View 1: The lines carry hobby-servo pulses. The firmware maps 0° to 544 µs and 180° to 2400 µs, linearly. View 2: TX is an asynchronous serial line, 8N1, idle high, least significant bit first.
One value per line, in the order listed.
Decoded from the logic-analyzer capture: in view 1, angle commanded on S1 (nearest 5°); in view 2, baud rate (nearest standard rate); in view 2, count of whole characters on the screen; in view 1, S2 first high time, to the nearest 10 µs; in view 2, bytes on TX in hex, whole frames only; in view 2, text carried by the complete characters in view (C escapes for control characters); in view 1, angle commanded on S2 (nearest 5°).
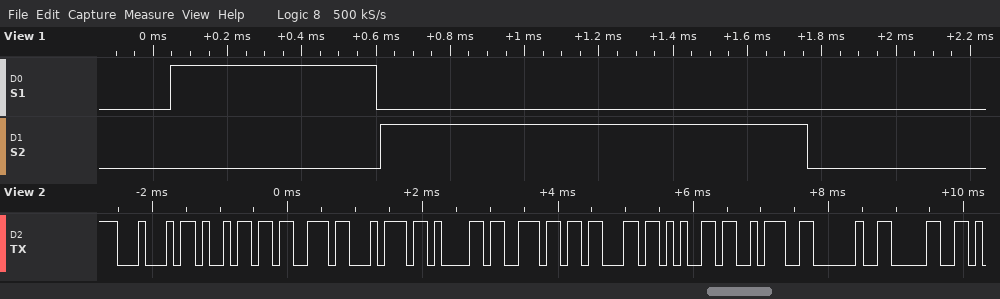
0°
9600 baud
11
1150 µs
0x44 0x69 0x73 0x74 0x61 0x6E 0x63 0x65 0x3A 0x20 0x30
"Distance: 0"
60°
